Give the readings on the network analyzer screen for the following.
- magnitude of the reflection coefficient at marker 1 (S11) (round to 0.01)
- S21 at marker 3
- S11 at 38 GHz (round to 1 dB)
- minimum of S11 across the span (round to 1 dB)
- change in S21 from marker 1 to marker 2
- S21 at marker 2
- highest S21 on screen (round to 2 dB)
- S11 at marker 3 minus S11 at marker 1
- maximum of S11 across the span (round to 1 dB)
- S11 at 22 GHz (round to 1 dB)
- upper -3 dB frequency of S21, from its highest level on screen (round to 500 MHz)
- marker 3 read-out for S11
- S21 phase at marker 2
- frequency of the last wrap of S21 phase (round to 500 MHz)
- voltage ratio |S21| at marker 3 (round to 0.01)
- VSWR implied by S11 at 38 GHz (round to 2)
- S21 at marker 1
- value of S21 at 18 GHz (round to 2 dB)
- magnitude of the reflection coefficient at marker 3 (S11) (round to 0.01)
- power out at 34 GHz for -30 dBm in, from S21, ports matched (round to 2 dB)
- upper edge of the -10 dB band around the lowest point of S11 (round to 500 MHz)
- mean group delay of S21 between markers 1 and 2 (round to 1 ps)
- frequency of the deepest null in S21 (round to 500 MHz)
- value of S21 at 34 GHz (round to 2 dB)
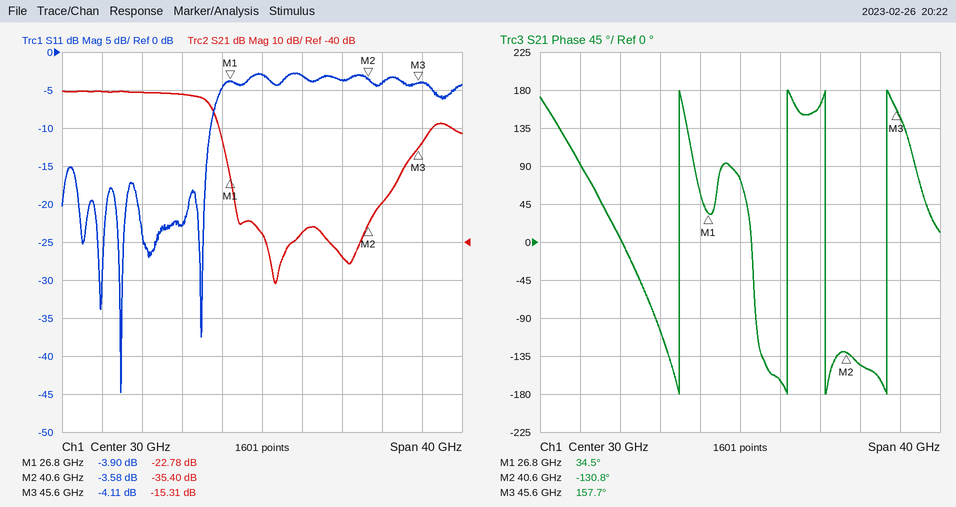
0.64
-15.31 dB
-4 dB
-45 dB
-12.62 dB
-35.40 dB
0 dB
-0.21 dB
-3 dB
-23 dB
24.5 GHz
-4.11 dB
-130.8°
44.5 GHz
0.17
4
-22.78 dB
0 dB
0.62
-68 dBm
25.0 GHz
33 ps
31.5 GHz
-38 dB
